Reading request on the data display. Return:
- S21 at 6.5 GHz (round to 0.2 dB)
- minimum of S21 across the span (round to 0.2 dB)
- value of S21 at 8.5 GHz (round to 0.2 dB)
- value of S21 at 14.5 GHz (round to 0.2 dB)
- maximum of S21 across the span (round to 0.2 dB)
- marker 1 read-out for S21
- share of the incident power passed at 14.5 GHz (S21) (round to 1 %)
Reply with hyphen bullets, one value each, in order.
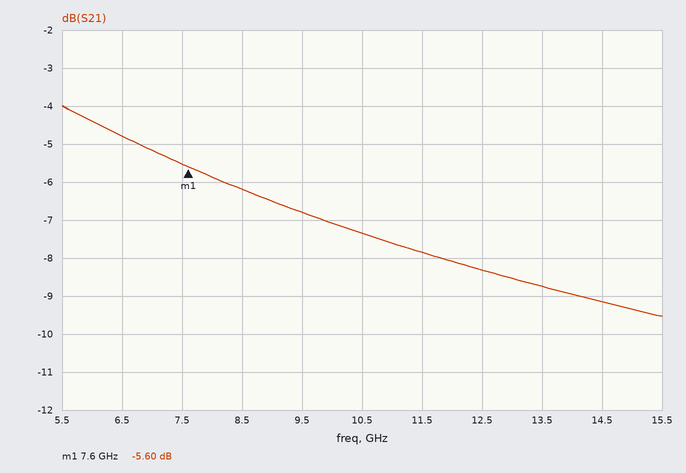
- -4.8 dB
- -9.6 dB
- -6.2 dB
- -9.2 dB
- -4.0 dB
- -5.60 dB
- 12 %
